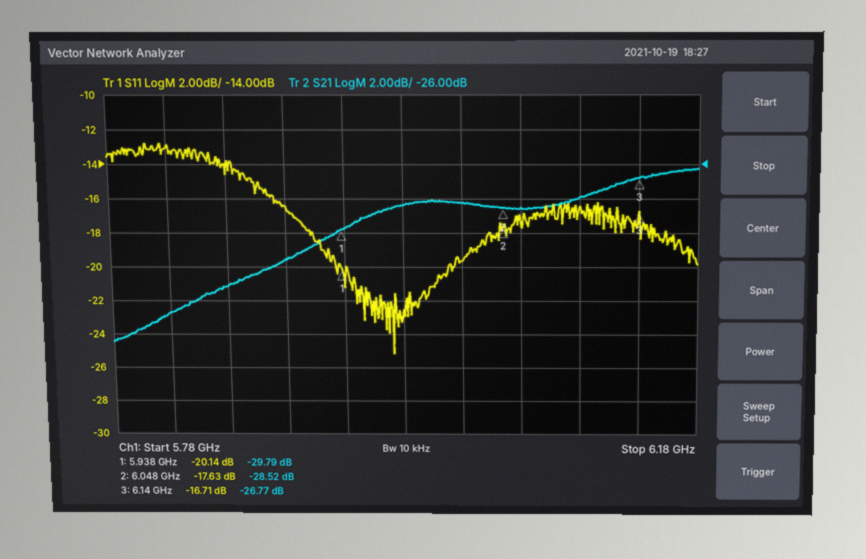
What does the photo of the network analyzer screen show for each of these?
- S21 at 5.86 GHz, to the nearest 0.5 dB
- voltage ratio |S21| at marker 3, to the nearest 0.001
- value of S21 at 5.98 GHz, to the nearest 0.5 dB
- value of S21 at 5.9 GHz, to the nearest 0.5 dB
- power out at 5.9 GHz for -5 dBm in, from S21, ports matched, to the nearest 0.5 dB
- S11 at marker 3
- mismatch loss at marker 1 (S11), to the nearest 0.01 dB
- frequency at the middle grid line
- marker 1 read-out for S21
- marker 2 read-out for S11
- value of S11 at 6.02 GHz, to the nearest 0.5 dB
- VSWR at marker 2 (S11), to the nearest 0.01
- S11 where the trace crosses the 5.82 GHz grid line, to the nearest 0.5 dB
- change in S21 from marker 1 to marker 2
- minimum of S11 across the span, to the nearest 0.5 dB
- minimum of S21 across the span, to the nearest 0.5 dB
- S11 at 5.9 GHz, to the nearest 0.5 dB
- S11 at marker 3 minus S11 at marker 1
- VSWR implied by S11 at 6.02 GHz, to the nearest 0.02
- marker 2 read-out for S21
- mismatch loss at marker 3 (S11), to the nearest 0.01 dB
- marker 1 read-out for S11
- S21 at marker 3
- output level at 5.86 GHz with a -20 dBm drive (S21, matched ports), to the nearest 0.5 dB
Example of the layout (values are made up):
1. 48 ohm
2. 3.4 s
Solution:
1. -33.0 dB
2. 0.046
3. -28.5 dB
4. -31.5 dB
5. -36.5 dBm
6. -16.71 dB
7. 0.04 dB
8. 5.98 GHz
9. -29.79 dB
10. -17.63 dB
11. -19.5 dB
12. 1.30
13. -13.0 dB
14. 1.27 dB
15. -25.0 dB
16. -36.5 dB
17. -16.5 dB
18. 3.43 dB
19. 1.24
20. -28.52 dB
21. 0.09 dB
22. -20.14 dB
23. -26.77 dB
24. -53.0 dBm
